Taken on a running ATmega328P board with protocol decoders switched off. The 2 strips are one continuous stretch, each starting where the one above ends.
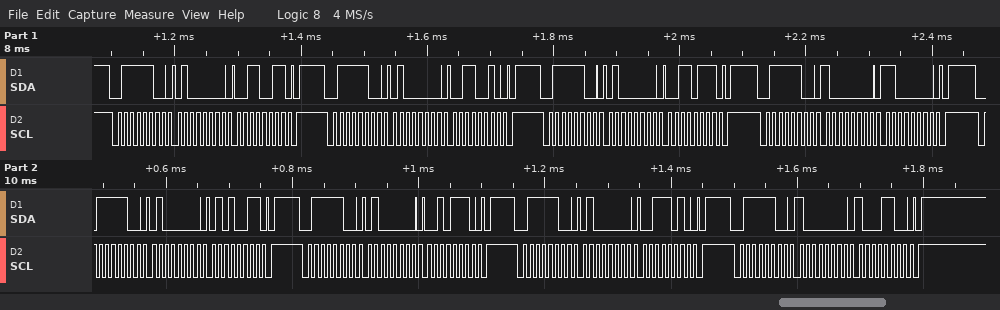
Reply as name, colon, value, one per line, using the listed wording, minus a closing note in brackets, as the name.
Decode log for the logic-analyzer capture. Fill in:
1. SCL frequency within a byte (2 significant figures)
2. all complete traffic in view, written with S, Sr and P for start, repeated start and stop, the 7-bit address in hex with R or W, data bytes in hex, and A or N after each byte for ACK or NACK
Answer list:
SCL frequency within a byte: 100 kHz
all complete traffic in view, written with S, Sr and P for start, repeated start and stop, the 7-bit address in hex with R or W, data bytes in hex, and A or N after each byte for ACK or NACK: S 3EW A 40 A 33 A P S 3EW A 40 A 32 A P S 3EW A 40 A 37 A P S 3EW A 80 A C0 A P S 3EW A 40 A 53 A P S 3EW A 40 A 2E A P S 3EW A 40 A 3A A P S 3EW A 80 A 8C A P
